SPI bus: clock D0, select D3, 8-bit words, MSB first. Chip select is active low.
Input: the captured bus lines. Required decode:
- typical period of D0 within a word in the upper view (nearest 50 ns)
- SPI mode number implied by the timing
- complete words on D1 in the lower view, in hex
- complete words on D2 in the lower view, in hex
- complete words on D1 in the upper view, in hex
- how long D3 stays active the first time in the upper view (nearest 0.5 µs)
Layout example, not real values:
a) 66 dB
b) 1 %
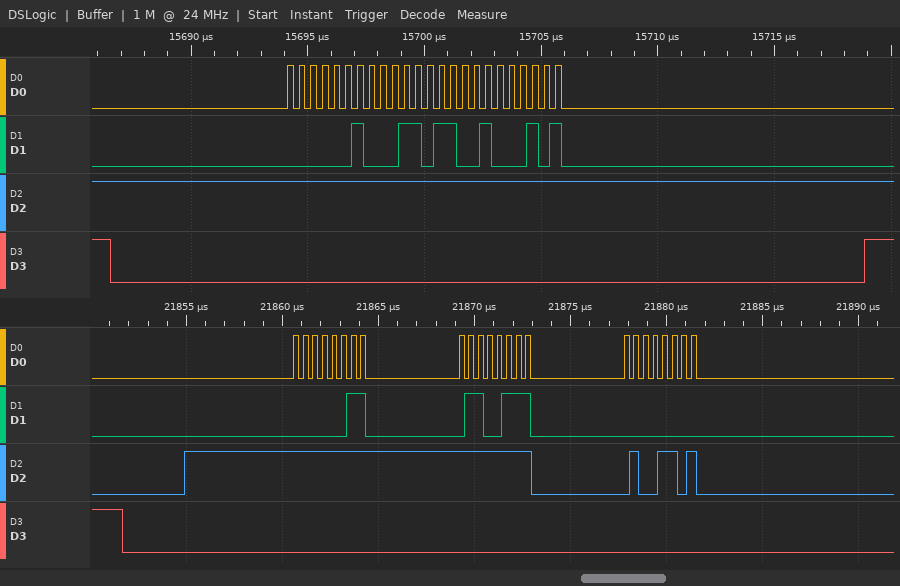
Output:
a) 500 ns
b) 0
c) 03, 67, 00
d) FF, FF, 4D
e) 02, 36, 45
f) 32.5 µs
